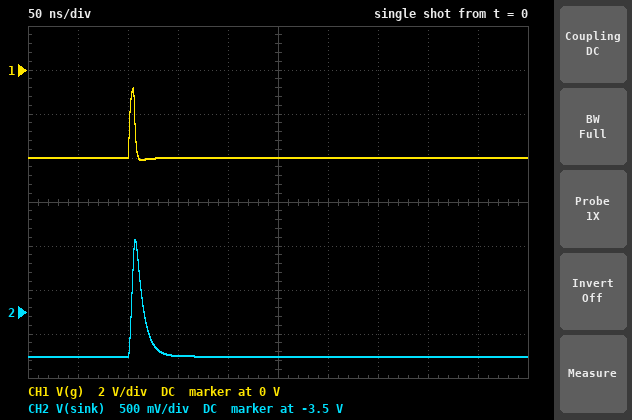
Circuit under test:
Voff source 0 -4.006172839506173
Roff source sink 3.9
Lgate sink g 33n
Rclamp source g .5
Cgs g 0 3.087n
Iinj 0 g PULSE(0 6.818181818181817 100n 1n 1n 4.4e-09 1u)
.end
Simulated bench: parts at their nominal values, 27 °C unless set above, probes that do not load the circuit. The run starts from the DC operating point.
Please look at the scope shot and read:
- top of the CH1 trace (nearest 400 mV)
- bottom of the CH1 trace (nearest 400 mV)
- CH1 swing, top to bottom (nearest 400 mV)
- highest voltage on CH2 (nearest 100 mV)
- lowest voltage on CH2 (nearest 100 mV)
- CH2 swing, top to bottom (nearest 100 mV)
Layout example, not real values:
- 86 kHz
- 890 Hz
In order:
- -800 mV
- -4.0 V
- 3.2 V
- -2.7 V
- -4.0 V
- 1.3 V
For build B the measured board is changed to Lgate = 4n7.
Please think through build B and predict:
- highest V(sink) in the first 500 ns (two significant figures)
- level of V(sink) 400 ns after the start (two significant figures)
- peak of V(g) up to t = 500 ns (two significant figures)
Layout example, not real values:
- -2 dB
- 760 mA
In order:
- -1.2 V
- -4.0 V
- -1.0 V
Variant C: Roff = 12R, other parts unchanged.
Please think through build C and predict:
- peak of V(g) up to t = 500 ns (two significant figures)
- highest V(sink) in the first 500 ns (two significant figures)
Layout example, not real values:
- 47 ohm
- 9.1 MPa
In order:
- -810 mV
- -1.6 V
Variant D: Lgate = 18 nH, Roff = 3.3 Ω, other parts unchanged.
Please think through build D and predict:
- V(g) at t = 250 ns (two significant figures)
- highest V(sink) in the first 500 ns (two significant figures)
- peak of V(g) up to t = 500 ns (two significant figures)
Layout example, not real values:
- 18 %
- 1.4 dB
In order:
- -4.0 V
- -2.3 V
- -890 mV
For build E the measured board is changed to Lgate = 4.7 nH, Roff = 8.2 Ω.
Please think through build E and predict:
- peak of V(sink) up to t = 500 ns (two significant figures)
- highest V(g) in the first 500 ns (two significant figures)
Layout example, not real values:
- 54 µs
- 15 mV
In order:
- -950 mV
- -890 mV
